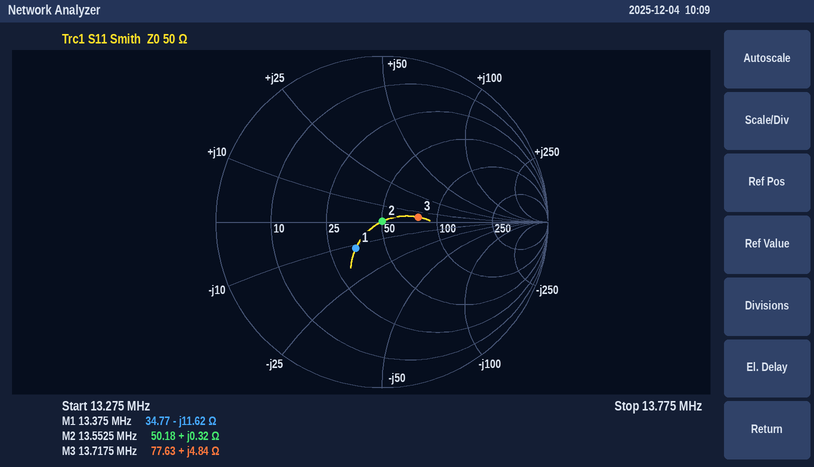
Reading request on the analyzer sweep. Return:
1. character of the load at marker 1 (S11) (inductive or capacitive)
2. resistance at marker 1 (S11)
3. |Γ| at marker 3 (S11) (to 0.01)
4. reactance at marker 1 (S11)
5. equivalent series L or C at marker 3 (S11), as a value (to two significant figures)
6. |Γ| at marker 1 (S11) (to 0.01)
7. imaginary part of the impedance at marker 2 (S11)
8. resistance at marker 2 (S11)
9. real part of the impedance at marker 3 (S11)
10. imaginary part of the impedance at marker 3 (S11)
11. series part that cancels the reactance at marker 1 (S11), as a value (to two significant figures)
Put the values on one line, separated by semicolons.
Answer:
capacitive; 34.77 Ω; 0.22; -11.62 Ω; 56 nH; 0.22; +0.32 Ω; 50.18 Ω; 77.63 Ω; +4.84 Ω; 140 nH
